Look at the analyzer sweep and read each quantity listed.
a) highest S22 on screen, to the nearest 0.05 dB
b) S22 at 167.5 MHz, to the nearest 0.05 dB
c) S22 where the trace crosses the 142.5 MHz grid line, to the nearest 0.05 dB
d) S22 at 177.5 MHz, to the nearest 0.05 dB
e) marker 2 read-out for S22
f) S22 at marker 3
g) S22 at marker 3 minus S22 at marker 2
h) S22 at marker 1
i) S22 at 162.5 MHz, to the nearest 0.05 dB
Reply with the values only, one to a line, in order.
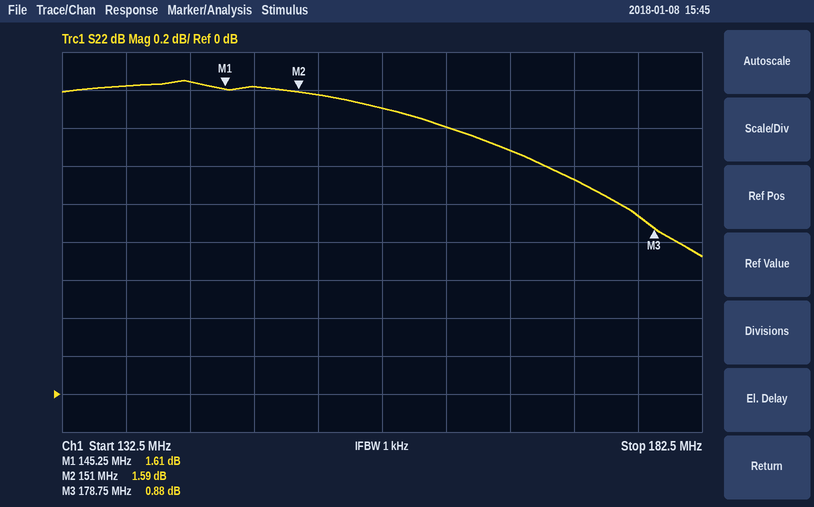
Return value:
1.65 dB
1.30 dB
1.65 dB
0.95 dB
1.59 dB
0.88 dB
-0.71 dB
1.61 dB
1.40 dB
